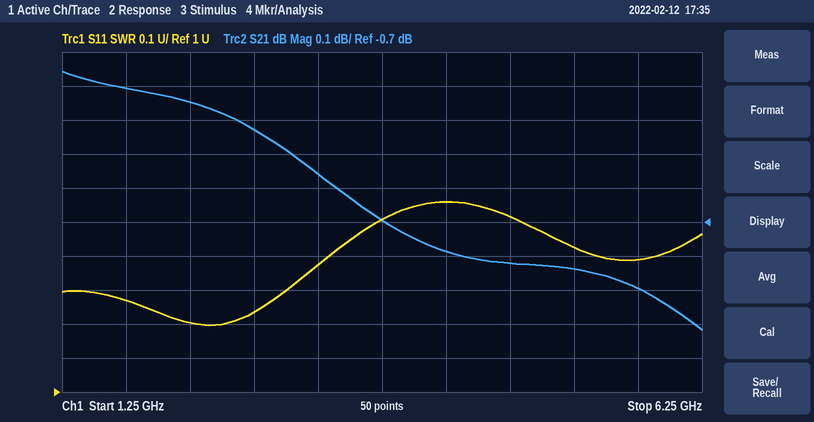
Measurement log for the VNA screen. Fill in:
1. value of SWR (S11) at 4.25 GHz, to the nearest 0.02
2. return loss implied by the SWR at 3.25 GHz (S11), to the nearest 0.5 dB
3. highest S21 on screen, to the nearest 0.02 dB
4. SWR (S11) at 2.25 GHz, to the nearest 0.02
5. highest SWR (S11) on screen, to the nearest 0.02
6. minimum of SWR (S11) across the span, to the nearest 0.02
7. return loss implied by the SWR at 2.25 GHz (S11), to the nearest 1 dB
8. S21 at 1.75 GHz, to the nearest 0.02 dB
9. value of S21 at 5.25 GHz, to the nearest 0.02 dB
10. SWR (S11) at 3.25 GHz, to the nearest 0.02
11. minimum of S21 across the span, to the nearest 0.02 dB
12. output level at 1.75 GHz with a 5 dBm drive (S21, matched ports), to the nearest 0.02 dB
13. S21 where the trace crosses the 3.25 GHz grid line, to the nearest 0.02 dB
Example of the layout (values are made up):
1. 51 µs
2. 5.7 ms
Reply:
1. 1.56
2. 16.0 dB
3. -0.26 dB
4. 1.20
5. 1.56
6. 1.20
7. 21 dB
8. -0.30 dB
9. -0.84 dB
10. 1.38
11. -1.02 dB
12. 4.70 dBm
13. -0.56 dB
